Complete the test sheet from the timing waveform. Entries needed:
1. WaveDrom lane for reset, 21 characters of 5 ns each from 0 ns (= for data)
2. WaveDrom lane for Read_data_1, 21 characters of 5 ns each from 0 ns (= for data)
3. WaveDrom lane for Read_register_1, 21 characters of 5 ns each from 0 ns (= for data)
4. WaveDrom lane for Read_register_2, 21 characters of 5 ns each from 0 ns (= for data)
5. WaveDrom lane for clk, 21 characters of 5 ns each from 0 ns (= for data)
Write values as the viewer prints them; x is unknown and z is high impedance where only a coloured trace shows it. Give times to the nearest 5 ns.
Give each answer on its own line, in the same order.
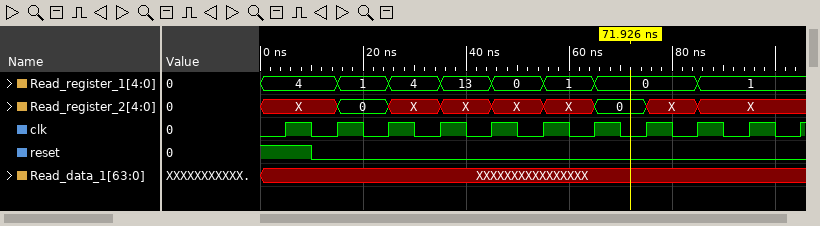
{name: 'reset', wave: '1.0..................'}
{name: 'Read_data_1', wave: 'x....................'}
{name: 'Read_register_1', wave: '=..=.=.=.=.=.=...=...', data: '4 1 4 13 0 1 0 1'}
{name: 'Read_register_2', wave: '=..=.=.=.=.=.=.=.x...', data: 'X 0 X X X X 0 X'}
{name: 'clk', wave: '010101010101010101010'}
